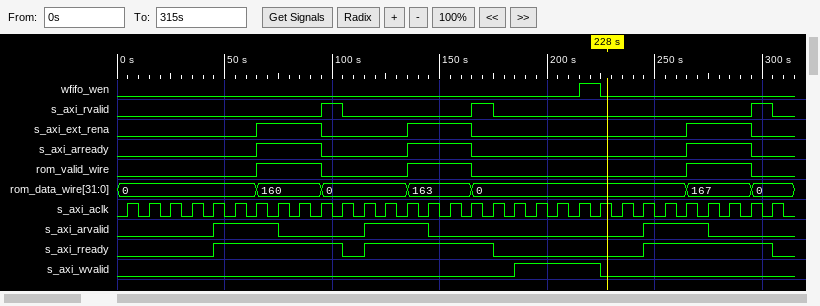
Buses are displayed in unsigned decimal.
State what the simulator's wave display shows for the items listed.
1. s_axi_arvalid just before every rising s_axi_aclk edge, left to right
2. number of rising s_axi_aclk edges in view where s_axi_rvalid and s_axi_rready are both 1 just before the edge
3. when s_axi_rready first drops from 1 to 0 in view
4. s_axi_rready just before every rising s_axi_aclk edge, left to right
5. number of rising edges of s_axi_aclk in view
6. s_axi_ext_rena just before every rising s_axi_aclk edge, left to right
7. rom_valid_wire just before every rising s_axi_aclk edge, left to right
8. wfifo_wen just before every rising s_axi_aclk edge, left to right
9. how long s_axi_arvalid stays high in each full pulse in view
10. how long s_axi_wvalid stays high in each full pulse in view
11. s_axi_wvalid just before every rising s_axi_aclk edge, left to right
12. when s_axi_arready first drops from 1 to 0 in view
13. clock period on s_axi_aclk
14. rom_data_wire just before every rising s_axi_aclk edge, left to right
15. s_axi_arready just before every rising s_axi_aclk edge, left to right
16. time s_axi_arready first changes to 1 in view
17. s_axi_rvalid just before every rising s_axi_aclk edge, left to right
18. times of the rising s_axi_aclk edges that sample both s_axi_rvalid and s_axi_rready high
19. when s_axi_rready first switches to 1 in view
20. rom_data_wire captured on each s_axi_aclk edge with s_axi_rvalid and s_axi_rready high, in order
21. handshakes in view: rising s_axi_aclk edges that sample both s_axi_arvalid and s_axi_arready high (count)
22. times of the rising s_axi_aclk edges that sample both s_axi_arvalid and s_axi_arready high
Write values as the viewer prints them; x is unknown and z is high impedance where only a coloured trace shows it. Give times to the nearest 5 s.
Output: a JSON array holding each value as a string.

["0 0 0 0 0 1 1 1 0 0 0 0 1 1 1 0 0 0 0 0 0 0 0 0 0 1 1 1 0 0 0", "3", "105 s", "0 0 0 0 0 1 1 1 1 1 1 0 1 1 1 1 1 1 0 0 0 0 0 0 0 1 1 1 1 1 1", "31", "0 0 0 0 0 0 0 1 1 1 0 0 0 0 1 1 1 0 0 0 0 0 0 0 0 0 0 1 1 1 0", "0 0 0 0 0 0 0 1 1 1 0 0 0 0 1 1 1 0 0 0 0 0 0 0 0 0 0 1 1 1 0", "0 0 0 0 0 0 0 0 0 0 0 0 0 0 0 0 0 0 0 0 0 0 1 0 0 0 0 0 0 0 0", "30 s, 30 s, 30 s", "40 s", "0 0 0 0 0 0 0 0 0 0 0 0 0 0 0 0 0 0 0 1 1 1 1 0 0 0 0 0 0 0 0", "95 s", "10 s", "0, 0, 0, 0, 0, 0, 0, 160, 160, 160, 0, 0, 0, 0, 163, 163, 163, 0, 0, 0, 0, 0, 0, 0, 0, 0, 0, 167, 167, 167, 0", "0 0 0 0 0 0 0 1 1 1 0 0 0 0 1 1 1 0 0 0 0 0 0 0 0 0 0 1 1 1 0", "65 s", "0 0 0 0 0 0 0 0 0 0 1 0 0 0 0 0 0 1 0 0 0 0 0 0 0 0 0 0 0 0 1", "105 s, 175 s, 305 s", "45 s", "0, 0, 0", "3", "75 s, 145 s, 275 s"]
